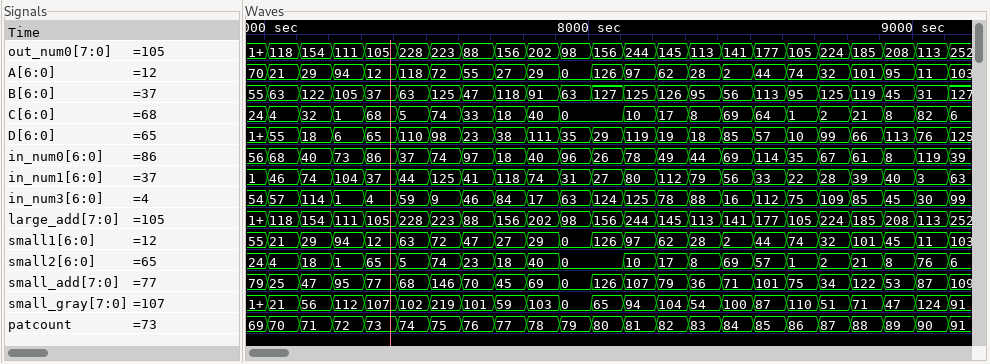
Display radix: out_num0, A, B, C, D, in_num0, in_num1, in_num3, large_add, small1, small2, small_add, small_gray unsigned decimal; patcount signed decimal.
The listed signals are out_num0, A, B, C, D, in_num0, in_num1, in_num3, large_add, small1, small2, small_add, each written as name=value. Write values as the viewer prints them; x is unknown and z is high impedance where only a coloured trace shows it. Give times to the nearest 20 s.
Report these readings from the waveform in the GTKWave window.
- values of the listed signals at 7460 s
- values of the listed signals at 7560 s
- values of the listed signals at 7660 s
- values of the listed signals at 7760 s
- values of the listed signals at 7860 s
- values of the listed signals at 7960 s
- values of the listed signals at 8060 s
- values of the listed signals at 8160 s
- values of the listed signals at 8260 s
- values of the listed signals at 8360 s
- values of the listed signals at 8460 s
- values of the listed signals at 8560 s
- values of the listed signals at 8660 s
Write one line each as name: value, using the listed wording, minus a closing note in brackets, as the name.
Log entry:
values of the listed signals at 7460 s: out_num0=228, A=118, B=63, C=5, D=110, in_num0=37, in_num1=44, in_num3=59, large_add=228, small1=63, small2=5, small_add=68
values of the listed signals at 7560 s: out_num0=223, A=72, B=125, C=74, D=98, in_num0=74, in_num1=125, in_num3=9, large_add=223, small1=72, small2=74, small_add=146
values of the listed signals at 7660 s: out_num0=88, A=55, B=47, C=33, D=23, in_num0=97, in_num1=41, in_num3=46, large_add=88, small1=47, small2=23, small_add=70
values of the listed signals at 7760 s: out_num0=156, A=27, B=118, C=18, D=38, in_num0=18, in_num1=118, in_num3=84, large_add=156, small1=27, small2=18, small_add=45
values of the listed signals at 7860 s: out_num0=202, A=29, B=91, C=40, D=111, in_num0=40, in_num1=74, in_num3=17, large_add=202, small1=29, small2=40, small_add=69
values of the listed signals at 7960 s: out_num0=98, A=0, B=63, C=0, D=35, in_num0=96, in_num1=31, in_num3=63, large_add=98, small1=0, small2=0, small_add=0
values of the listed signals at 8060 s: out_num0=156, A=126, B=127, C=0, D=29, in_num0=26, in_num1=27, in_num3=124, large_add=156, small1=126, small2=0, small_add=126
values of the listed signals at 8160 s: out_num0=244, A=97, B=125, C=10, D=119, in_num0=78, in_num1=80, in_num3=125, large_add=244, small1=97, small2=10, small_add=107
values of the listed signals at 8260 s: out_num0=145, A=62, B=126, C=17, D=19, in_num0=49, in_num1=112, in_num3=78, large_add=145, small1=62, small2=17, small_add=79
values of the listed signals at 8360 s: out_num0=113, A=28, B=95, C=8, D=18, in_num0=44, in_num1=79, in_num3=88, large_add=113, small1=28, small2=8, small_add=36
values of the listed signals at 8460 s: out_num0=141, A=2, B=56, C=69, D=85, in_num0=69, in_num1=56, in_num3=16, large_add=141, small1=2, small2=69, small_add=71
values of the listed signals at 8560 s: out_num0=177, A=44, B=113, C=64, D=57, in_num0=114, in_num1=33, in_num3=112, large_add=177, small1=44, small2=57, small_add=101
values of the listed signals at 8660 s: out_num0=105, A=74, B=95, C=1, D=10, in_num0=35, in_num1=22, in_num3=75, large_add=105, small1=74, small2=1, small_add=75
